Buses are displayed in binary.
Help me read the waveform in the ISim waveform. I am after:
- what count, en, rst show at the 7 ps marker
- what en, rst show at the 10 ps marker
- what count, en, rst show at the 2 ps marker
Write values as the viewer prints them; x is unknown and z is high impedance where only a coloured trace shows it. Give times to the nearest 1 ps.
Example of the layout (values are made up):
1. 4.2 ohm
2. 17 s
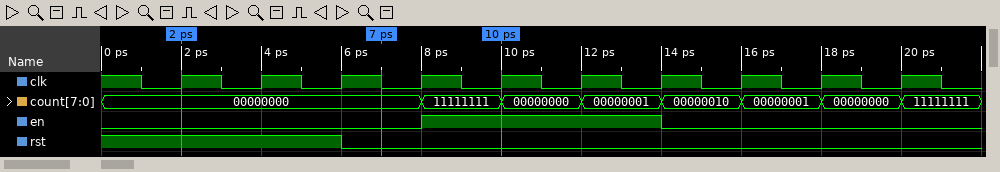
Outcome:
1. count=00000000, en=0, rst=0
2. en=1, rst=0
3. count=00000000, en=0, rst=1
